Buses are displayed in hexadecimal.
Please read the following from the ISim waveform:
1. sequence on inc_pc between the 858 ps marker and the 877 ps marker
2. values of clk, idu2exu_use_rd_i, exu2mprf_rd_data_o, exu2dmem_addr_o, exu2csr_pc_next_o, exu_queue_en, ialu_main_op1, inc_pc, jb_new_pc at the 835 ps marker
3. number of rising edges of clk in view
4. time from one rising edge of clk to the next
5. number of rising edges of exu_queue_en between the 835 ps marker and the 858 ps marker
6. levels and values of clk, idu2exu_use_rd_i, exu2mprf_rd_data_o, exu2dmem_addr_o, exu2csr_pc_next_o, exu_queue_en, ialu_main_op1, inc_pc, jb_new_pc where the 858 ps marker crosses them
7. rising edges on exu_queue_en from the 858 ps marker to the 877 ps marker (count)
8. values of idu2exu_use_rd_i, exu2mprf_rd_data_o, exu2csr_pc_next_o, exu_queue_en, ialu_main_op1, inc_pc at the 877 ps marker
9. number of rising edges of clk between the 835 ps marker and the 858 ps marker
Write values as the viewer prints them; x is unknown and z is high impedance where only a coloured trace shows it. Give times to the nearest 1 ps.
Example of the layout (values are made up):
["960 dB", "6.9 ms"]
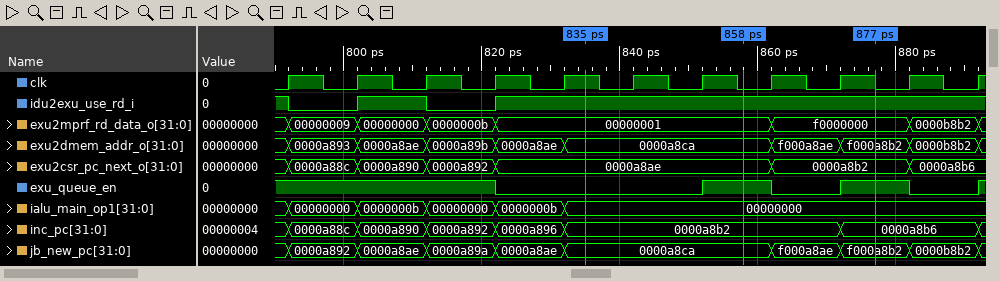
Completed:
["0000a8b2, 0000a8b6", "clk=1, idu2exu_use_rd_i=1, exu2mprf_rd_data_o=00000001, exu2dmem_addr_o=0000a8ca, exu2csr_pc_next_o=0000a8ae, exu_queue_en=0, ialu_main_op1=00000000, inc_pc=0000a8b2, jb_new_pc=0000a8ca", "11", "10 ps", "1", "clk=0, idu2exu_use_rd_i=1, exu2mprf_rd_data_o=00000001, exu2dmem_addr_o=0000a8ca, exu2csr_pc_next_o=0000a8ae, exu_queue_en=1, ialu_main_op1=00000000, inc_pc=0000a8b2, jb_new_pc=0000a8ca", "1", "idu2exu_use_rd_i=1, exu2mprf_rd_data_o=f0000000, exu2csr_pc_next_o=0000a8b2, exu_queue_en=1, ialu_main_op1=00000000, inc_pc=0000a8b6", "2"]
